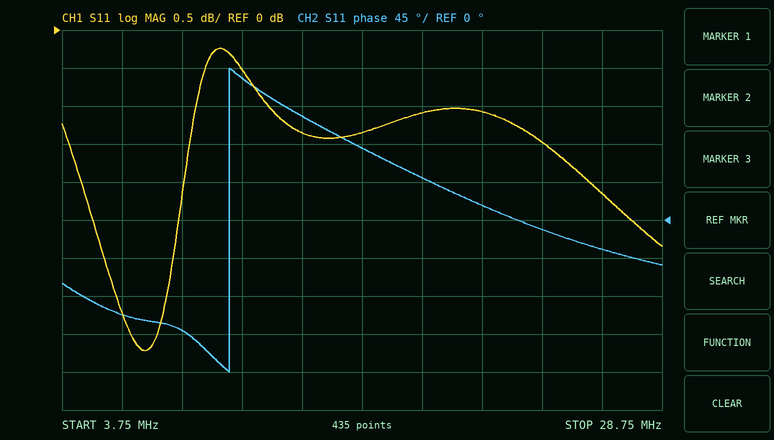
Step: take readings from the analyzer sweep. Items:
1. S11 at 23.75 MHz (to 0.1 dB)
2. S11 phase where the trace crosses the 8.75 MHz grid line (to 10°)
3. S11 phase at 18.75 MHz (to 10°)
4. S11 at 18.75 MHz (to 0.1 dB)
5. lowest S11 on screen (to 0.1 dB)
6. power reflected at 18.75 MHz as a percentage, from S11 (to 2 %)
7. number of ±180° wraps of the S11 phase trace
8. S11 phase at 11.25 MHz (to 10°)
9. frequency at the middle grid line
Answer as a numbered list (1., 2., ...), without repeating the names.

1. -1.5 dB
2. -130°
3. 50°
4. -1.1 dB
5. -4.2 dB
6. 78 %
7. 1
8. 170°
9. 16.25 MHz
